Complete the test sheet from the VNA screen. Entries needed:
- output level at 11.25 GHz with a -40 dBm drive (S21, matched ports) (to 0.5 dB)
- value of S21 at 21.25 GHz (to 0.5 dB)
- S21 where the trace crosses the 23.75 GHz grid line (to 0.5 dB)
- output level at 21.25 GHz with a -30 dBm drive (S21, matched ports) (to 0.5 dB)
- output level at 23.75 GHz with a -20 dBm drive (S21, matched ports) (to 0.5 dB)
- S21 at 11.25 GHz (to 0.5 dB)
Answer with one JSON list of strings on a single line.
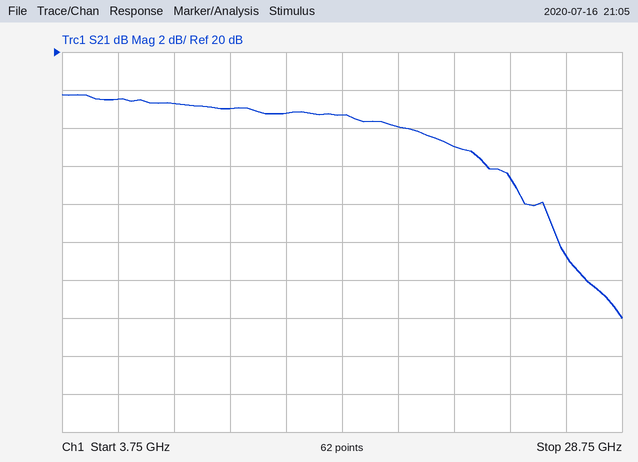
["-23.0 dBm", "15.0 dB", "13.5 dB", "-15.0 dBm", "-6.5 dBm", "17.0 dB"]
